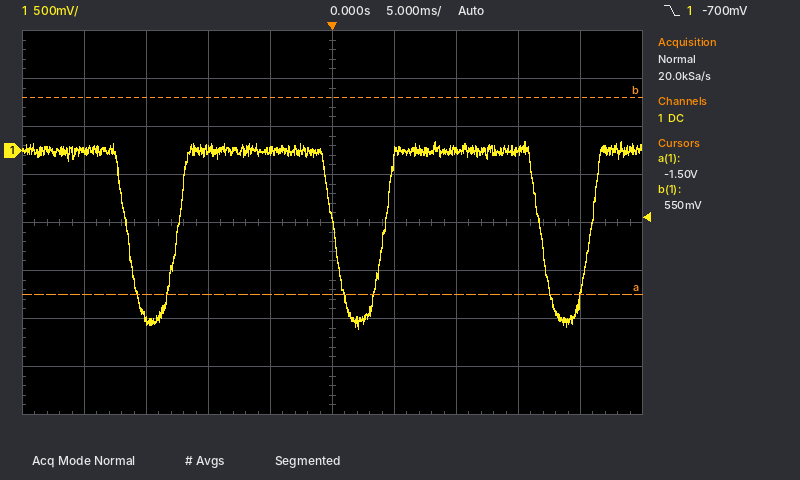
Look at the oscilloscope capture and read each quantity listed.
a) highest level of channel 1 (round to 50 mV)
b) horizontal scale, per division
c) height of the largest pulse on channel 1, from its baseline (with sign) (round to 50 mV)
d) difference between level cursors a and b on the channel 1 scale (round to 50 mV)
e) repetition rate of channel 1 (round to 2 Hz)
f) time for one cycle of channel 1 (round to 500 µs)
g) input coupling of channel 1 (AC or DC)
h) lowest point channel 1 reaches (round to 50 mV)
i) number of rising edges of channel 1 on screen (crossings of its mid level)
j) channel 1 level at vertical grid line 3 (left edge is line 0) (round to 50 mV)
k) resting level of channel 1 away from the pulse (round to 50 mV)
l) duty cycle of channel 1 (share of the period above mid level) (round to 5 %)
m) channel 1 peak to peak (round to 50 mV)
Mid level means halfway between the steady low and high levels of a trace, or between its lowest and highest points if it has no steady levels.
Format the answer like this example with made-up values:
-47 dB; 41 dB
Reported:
100 mV; 5 ms; -1.85 V; 2.05 V; 60 Hz; 16.5 ms; DC; -1.85 V; 3; 0 mV; 0 mV; 75 %; 1.95 V
